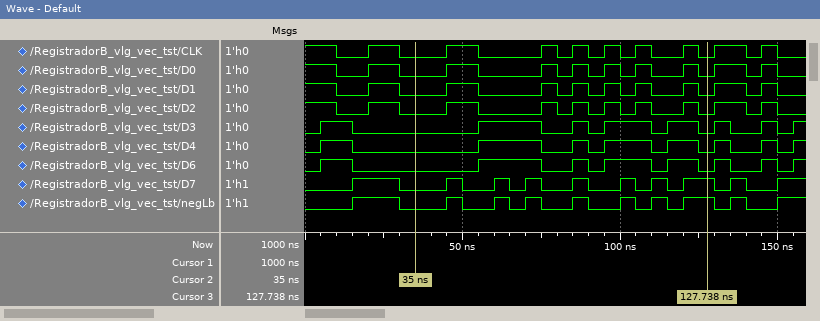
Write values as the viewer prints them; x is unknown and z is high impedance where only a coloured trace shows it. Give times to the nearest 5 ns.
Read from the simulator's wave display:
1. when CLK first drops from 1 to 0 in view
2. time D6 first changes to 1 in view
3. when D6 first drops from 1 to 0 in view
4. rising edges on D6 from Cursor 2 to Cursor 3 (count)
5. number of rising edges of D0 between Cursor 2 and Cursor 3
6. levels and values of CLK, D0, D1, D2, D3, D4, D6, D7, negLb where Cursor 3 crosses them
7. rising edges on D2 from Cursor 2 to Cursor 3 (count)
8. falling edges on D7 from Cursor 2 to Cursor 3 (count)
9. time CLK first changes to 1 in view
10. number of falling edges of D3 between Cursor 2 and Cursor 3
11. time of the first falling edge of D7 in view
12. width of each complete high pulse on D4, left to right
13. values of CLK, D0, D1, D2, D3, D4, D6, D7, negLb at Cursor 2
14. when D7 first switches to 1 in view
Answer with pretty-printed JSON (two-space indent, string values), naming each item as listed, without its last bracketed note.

{
  "when CLK first drops from 1 to 0 in view": "10 ns",
  "time D6 first changes to 1 in view": "5 ns",
  "when D6 first drops from 1 to 0 in view": "15 ns",
  "rising edges on D6 from Cursor 2 to Cursor 3": "4",
  "number of rising edges of D0 between Cursor 2 and Cursor 3": "6",
  "levels and values of CLK, D0, D1, D2, D3, D4, D6, D7, negLb where Cursor 3 crosses them": "CLK=0, D0=0, D1=0, D2=0, D3=0, D4=0, D6=0, D7=1, negLb=1",
  "rising edges on D2 from Cursor 2 to Cursor 3": "6",
  "falling edges on D7 from Cursor 2 to Cursor 3": "6",
  "time CLK first changes to 1 in view": "20 ns",
  "number of falling edges of D3 between Cursor 2 and Cursor 3": "4",
  "time of the first falling edge of D7 in view": "30 ns",
  "width of each complete high pulse on D4, left to right": "10 ns, 20 ns, 5 ns, 15 ns, 10 ns, 5 ns, 5 ns",
  "values of CLK, D0, D1, D2, D3, D4, D6, D7, negLb at Cursor 2": "CLK=0, D0=0, D1=0, D2=0, D3=0, D4=0, D6=0, D7=0, negLb=0",
  "when D7 first switches to 1 in view": "15 ns"
}
